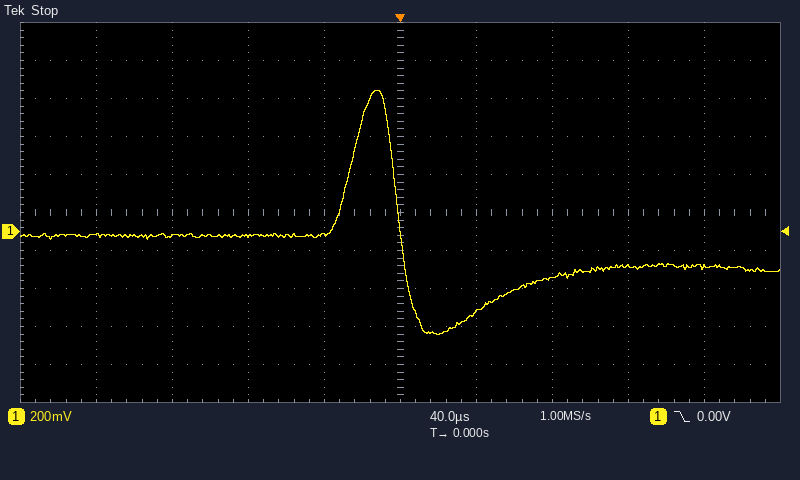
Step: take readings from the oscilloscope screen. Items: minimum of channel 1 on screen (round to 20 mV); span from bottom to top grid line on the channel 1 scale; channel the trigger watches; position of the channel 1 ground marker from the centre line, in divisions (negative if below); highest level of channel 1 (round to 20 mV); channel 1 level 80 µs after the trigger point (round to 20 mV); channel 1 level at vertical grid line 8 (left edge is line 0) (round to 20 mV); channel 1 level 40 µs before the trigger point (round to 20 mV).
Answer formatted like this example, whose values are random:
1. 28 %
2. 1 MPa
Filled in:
1. -540 mV
2. 2 V
3. channel 1
4. -0.5 div
5. 740 mV
6. -240 mV
7. -180 mV
8. -20 mV
